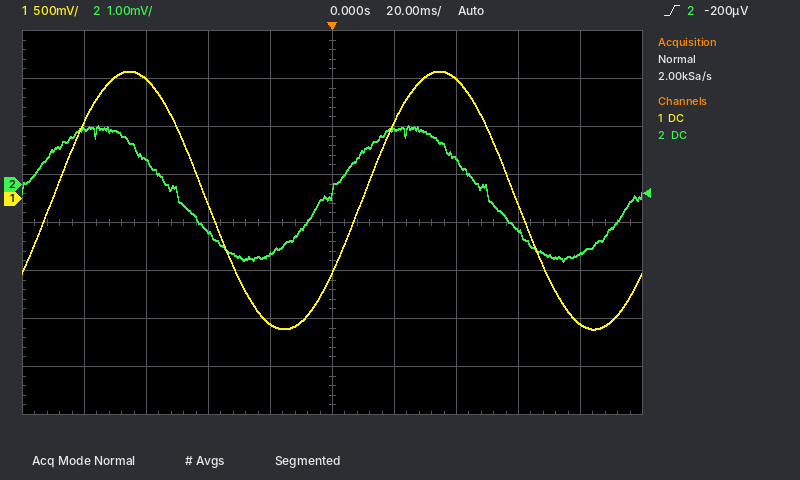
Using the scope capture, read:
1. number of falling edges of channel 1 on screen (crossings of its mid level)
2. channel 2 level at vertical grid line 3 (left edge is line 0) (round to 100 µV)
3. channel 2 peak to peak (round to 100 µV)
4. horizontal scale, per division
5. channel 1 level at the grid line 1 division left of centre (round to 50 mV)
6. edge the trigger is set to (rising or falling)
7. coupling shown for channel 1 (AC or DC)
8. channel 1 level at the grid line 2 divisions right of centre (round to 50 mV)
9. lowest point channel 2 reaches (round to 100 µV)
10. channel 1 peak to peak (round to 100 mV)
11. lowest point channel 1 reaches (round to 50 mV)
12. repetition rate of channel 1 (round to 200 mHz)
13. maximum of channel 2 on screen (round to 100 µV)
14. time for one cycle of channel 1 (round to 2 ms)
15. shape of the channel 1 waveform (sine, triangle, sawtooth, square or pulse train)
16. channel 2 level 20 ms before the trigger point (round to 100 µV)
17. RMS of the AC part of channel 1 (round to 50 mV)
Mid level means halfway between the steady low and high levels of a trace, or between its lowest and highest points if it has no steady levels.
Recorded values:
2
-1.0 mV
2.8 mV
20 ms
-1.30 V
rising
DC
1.25 V
-1.6 mV
2.70 V
-1.35 V
10.0 Hz
1.2 mV
100 ms
sine
-1.5 mV
950 mV
